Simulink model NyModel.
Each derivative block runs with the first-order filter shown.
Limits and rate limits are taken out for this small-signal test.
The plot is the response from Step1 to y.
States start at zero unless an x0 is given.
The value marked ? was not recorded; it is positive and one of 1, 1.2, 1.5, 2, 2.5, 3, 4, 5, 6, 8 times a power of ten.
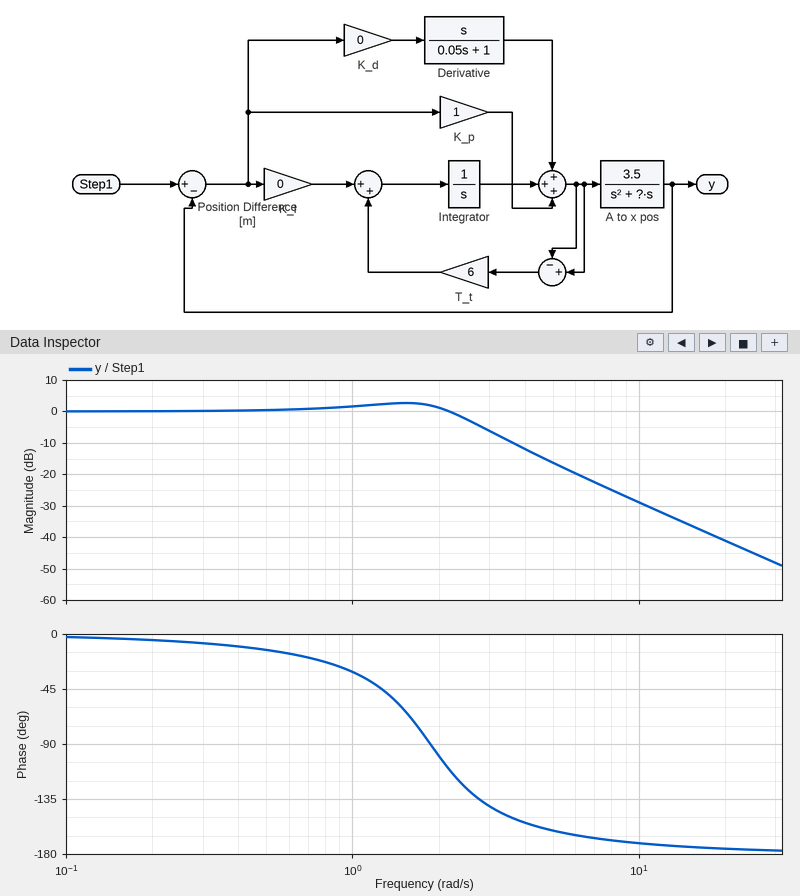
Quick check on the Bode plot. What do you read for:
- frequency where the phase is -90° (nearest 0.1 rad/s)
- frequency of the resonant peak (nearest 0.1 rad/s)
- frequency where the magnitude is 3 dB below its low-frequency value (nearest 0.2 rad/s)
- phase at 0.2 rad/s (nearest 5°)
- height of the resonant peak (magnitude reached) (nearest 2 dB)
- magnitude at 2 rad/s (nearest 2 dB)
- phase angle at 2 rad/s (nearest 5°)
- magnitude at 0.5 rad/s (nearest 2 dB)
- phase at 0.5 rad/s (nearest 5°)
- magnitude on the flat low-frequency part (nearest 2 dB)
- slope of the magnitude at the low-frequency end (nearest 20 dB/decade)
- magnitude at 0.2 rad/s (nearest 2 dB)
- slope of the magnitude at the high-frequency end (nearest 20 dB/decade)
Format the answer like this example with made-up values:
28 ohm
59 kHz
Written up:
1.9 rad/s
1.5 rad/s
2.6 rad/s
-5°
2 dB
2 dB
-100°
0 dB
-15°
0 dB
0 dB/decade
0 dB
-40 dB/decade
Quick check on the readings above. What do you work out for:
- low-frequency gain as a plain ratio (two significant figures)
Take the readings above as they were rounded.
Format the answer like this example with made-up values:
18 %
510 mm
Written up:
1.0
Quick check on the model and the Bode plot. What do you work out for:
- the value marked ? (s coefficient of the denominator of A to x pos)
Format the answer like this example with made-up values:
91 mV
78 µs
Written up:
1.5
